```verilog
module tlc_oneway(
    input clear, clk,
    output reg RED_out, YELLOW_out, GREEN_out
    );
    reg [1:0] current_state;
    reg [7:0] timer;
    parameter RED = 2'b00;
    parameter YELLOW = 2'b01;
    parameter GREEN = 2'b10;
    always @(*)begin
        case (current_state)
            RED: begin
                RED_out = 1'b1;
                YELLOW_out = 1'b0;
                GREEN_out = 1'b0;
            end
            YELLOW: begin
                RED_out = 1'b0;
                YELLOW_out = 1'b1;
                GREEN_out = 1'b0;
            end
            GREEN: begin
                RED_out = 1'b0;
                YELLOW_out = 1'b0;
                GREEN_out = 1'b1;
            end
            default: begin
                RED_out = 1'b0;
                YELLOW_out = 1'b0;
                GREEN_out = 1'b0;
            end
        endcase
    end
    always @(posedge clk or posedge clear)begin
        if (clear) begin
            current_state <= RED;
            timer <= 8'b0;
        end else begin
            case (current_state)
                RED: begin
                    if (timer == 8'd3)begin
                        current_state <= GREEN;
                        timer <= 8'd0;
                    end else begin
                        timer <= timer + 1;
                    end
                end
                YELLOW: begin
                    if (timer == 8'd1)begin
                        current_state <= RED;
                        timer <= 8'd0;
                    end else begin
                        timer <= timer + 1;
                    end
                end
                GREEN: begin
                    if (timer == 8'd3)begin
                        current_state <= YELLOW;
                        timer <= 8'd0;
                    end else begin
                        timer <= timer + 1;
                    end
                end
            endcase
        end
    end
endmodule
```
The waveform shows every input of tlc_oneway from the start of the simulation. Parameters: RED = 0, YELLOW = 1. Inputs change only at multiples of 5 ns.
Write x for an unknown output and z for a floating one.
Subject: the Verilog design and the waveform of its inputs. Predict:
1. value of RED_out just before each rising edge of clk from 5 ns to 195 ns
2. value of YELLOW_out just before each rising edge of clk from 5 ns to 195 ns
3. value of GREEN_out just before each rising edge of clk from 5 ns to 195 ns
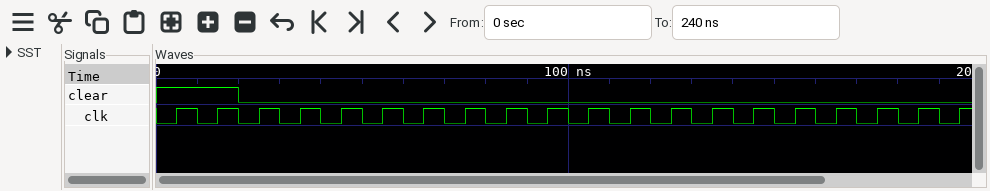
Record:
1 1 1 1 1 1 0 0 0 0 0 0 1 1 1 1 0 0 0 0
0 0 0 0 0 0 0 0 0 0 1 1 0 0 0 0 0 0 0 0
0 0 0 0 0 0 1 1 1 1 0 0 0 0 0 0 1 1 1 1
